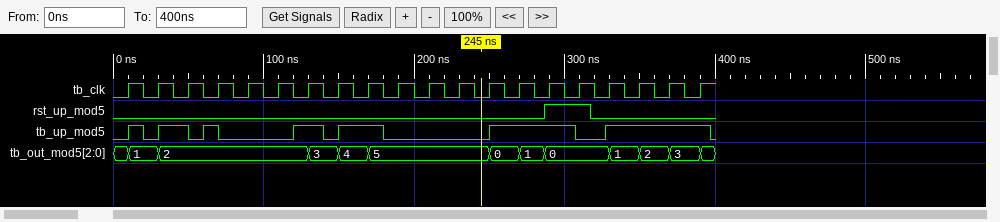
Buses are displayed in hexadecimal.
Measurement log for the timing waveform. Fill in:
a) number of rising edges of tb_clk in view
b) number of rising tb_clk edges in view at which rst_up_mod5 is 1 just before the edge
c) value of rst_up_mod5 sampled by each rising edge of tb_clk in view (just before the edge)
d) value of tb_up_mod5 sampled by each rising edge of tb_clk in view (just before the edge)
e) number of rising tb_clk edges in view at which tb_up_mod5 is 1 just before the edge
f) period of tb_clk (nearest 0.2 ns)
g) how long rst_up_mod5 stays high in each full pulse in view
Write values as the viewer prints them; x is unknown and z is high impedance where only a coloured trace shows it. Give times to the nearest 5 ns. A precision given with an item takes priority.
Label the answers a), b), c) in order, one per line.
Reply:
a) 20
b) 2
c) 0 0 0 0 0 0 0 0 0 0 0 0 0 0 1 1 0 0 0 0
d) 0 0 1 1 0 0 1 0 1 0 0 0 0 1 1 0 1 1 1 1
e) 10
f) 20 ns
g) 30 ns
